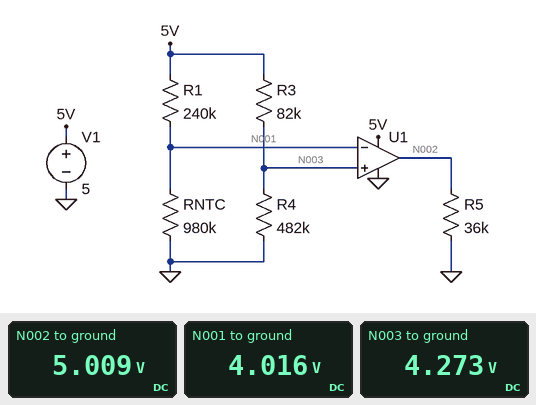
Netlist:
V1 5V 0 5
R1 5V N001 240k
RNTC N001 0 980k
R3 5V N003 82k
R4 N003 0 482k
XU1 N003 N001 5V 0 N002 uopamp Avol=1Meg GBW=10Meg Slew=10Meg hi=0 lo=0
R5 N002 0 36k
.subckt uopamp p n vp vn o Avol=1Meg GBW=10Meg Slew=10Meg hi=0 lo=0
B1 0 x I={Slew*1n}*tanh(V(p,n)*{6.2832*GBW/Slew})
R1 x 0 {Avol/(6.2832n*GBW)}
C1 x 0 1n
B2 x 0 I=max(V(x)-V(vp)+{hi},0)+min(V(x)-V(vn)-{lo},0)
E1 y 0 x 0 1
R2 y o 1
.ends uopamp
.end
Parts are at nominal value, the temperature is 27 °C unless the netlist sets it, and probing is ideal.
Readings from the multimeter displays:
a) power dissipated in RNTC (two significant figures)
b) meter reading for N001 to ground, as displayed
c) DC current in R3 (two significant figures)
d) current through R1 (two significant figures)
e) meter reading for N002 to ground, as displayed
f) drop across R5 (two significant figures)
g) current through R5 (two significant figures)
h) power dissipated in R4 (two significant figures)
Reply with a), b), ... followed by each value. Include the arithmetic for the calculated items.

a) (4.016 V)^2 / 980 kΩ = 16 µW
b) 4.016 V
c) (5 V - 4.273 V) / 82 kΩ = 8.9 µA
d) (5 V - 4.016 V) / 240 kΩ = 4.1 µA
e) 5.009 V
f) 5.009 V = 5.0 V
g) (5.009 V) / 36 kΩ = 140 µA
h) (4.273 V)^2 / 482 kΩ = 38 µW
